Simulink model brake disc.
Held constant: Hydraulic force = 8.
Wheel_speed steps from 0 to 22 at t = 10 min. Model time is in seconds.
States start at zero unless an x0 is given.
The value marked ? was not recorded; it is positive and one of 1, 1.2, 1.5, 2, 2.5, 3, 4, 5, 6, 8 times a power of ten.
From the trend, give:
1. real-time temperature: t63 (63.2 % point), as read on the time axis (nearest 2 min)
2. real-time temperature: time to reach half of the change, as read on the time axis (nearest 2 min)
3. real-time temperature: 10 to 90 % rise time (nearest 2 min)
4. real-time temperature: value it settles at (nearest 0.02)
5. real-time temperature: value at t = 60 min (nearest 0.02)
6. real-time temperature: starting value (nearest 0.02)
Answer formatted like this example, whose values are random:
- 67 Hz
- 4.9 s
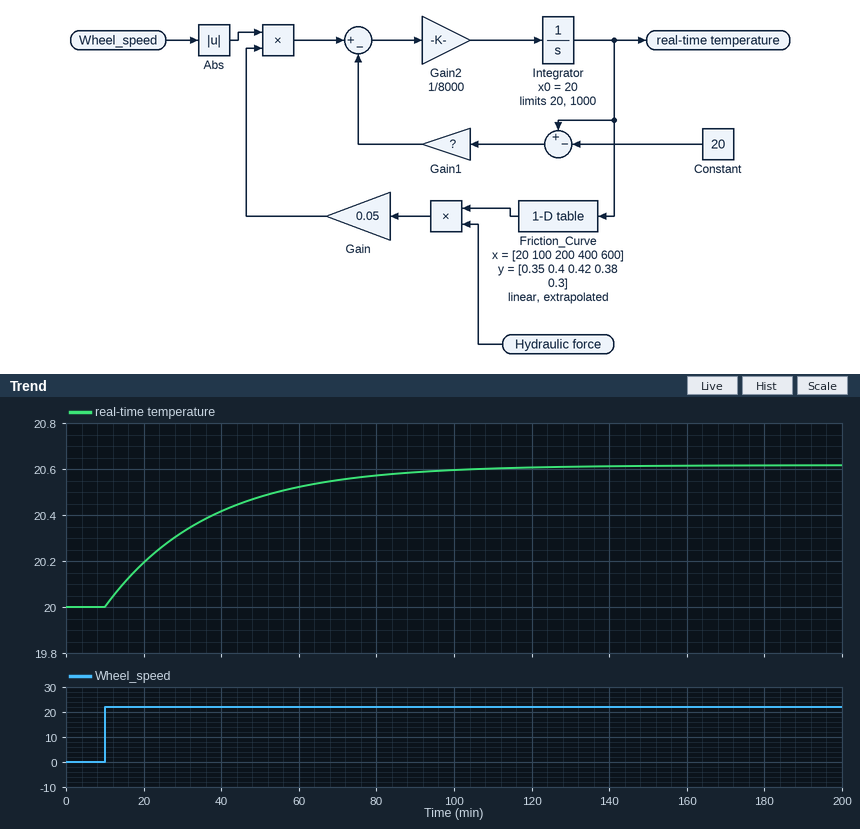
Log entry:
- 36 min
- 28 min
- 58 min
- 20.62
- 20.52
- 20.00
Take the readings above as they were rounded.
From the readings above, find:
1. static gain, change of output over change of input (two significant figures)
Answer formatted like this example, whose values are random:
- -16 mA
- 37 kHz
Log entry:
- 0.028
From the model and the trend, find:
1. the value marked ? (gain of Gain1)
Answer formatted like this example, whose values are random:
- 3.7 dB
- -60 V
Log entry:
- 5
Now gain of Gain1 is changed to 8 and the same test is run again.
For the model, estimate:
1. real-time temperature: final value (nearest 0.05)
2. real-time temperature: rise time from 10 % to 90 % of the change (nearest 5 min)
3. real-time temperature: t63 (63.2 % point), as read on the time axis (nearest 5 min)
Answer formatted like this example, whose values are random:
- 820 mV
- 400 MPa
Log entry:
- 20.40
- 35 min
- 25 min
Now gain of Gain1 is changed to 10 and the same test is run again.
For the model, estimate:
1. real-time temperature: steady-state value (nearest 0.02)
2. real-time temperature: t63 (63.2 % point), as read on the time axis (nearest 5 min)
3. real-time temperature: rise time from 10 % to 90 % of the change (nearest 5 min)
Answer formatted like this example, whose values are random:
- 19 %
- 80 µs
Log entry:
- 20.30
- 25 min
- 30 min
